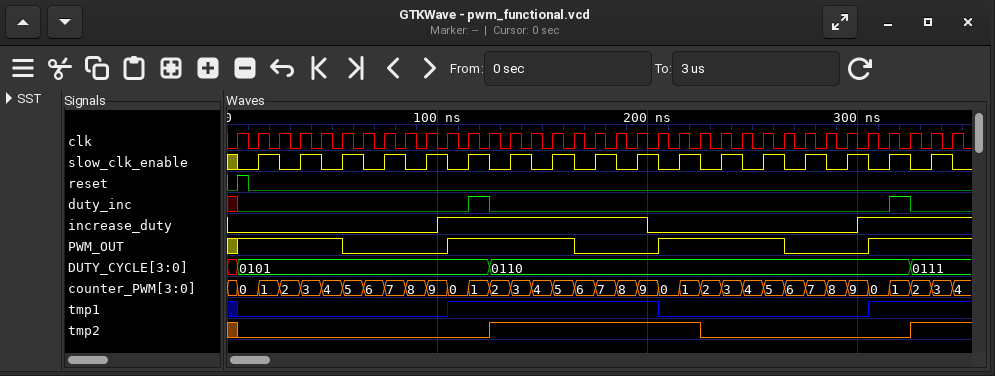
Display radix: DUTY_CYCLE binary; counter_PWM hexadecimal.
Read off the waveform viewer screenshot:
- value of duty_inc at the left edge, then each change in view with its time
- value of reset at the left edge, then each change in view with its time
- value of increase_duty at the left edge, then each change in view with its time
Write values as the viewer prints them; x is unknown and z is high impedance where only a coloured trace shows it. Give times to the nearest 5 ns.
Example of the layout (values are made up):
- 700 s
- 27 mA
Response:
- x, 0 at 5 ns, 1 at 115 ns, 0 at 125 ns, 1 at 315 ns, 0 at 325 ns
- 0, 1 at 5 ns, 0 at 10 ns
- 0, 1 at 100 ns, 0 at 200 ns, 1 at 300 ns
